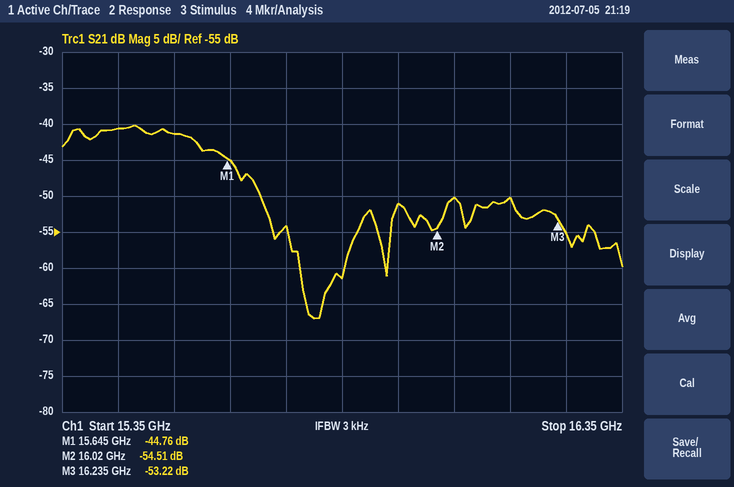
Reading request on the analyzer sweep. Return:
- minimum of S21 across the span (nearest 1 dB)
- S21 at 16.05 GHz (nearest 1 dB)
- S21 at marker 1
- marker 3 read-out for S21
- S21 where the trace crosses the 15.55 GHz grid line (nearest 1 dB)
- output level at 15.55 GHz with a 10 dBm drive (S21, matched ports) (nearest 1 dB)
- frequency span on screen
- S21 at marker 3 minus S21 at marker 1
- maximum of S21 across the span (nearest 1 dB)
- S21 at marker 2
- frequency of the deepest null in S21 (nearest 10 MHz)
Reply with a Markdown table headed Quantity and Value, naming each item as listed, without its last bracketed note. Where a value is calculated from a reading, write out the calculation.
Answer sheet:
| Quantity | Value |
|---|---|
| minimum of S21 across the span | -67 dB |
| S21 at 16.05 GHz | -50 dB |
| S21 at marker 1 | -44.76 dB |
| marker 3 read-out for S21 | -53.22 dB |
| S21 where the trace crosses the 15.55 GHz grid line | -41 dB |
| output level at 15.55 GHz with a 10 dBm drive (S21, matched ports) | 10 dBm + (-41 dB) = -31 dBm |
| frequency span on screen | 1 GHz |
| S21 at marker 3 minus S21 at marker 1 | -53.22 − (-44.76) = -8.46 dB |
| maximum of S21 across the span | -40 dB |
| S21 at marker 2 | -54.51 dB |
| frequency of the deepest null in S21 | 15.80 GHz |
